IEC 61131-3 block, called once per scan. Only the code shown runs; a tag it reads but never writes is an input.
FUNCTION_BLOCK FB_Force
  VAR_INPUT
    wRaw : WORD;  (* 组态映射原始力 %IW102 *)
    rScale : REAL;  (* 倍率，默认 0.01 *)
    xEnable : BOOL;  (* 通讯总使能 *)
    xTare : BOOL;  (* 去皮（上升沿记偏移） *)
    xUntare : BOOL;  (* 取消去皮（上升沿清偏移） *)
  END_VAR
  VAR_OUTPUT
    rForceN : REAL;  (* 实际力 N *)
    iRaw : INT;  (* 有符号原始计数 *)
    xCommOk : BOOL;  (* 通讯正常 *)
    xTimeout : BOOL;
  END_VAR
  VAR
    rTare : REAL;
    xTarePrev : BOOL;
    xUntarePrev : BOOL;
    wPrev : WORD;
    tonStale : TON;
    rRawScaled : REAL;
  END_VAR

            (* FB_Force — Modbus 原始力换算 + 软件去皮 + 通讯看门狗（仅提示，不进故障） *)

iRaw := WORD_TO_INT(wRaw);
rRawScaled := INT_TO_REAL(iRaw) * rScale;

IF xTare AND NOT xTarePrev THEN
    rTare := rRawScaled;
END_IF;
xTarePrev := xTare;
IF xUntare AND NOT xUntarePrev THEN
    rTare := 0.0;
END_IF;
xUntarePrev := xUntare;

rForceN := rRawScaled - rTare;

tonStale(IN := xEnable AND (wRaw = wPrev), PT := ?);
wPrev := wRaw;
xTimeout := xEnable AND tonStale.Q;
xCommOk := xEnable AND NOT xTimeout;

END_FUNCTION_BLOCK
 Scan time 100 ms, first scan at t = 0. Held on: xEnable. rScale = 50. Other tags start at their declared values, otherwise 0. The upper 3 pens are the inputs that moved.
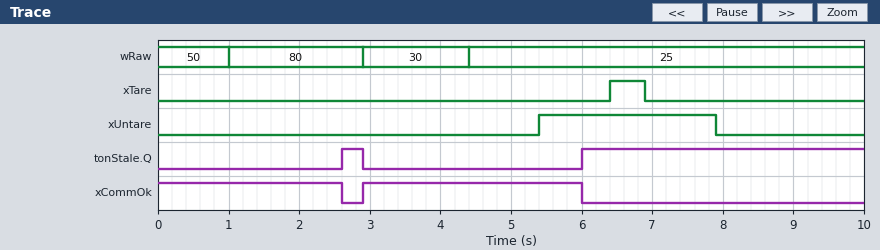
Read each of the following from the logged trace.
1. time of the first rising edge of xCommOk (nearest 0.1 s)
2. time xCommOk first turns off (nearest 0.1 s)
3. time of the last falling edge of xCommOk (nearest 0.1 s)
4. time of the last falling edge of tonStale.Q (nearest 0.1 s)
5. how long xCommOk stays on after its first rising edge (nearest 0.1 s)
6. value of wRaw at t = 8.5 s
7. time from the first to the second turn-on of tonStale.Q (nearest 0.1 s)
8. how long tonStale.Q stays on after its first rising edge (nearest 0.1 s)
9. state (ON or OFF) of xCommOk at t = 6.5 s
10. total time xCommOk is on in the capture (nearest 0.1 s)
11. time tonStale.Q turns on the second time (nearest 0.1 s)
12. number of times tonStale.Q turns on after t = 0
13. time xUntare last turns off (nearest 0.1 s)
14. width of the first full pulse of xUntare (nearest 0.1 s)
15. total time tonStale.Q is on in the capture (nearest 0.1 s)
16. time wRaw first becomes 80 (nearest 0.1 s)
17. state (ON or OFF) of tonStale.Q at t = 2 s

2.9 s
2.6 s
6.0 s
2.9 s
3.1 s
25
3.4 s
0.3 s
OFF
5.7 s
6.0 s
2
7.9 s
2.5 s
4.3 s
1.0 s
OFF
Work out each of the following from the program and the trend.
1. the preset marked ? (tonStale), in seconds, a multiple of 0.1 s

1.5 s
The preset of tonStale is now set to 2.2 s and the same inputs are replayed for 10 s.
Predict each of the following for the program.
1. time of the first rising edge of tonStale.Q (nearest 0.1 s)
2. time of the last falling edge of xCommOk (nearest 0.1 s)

6.7 s
6.7 s
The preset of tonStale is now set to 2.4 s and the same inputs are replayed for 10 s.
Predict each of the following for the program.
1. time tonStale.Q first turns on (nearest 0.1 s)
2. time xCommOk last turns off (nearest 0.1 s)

6.9 s
6.9 s
